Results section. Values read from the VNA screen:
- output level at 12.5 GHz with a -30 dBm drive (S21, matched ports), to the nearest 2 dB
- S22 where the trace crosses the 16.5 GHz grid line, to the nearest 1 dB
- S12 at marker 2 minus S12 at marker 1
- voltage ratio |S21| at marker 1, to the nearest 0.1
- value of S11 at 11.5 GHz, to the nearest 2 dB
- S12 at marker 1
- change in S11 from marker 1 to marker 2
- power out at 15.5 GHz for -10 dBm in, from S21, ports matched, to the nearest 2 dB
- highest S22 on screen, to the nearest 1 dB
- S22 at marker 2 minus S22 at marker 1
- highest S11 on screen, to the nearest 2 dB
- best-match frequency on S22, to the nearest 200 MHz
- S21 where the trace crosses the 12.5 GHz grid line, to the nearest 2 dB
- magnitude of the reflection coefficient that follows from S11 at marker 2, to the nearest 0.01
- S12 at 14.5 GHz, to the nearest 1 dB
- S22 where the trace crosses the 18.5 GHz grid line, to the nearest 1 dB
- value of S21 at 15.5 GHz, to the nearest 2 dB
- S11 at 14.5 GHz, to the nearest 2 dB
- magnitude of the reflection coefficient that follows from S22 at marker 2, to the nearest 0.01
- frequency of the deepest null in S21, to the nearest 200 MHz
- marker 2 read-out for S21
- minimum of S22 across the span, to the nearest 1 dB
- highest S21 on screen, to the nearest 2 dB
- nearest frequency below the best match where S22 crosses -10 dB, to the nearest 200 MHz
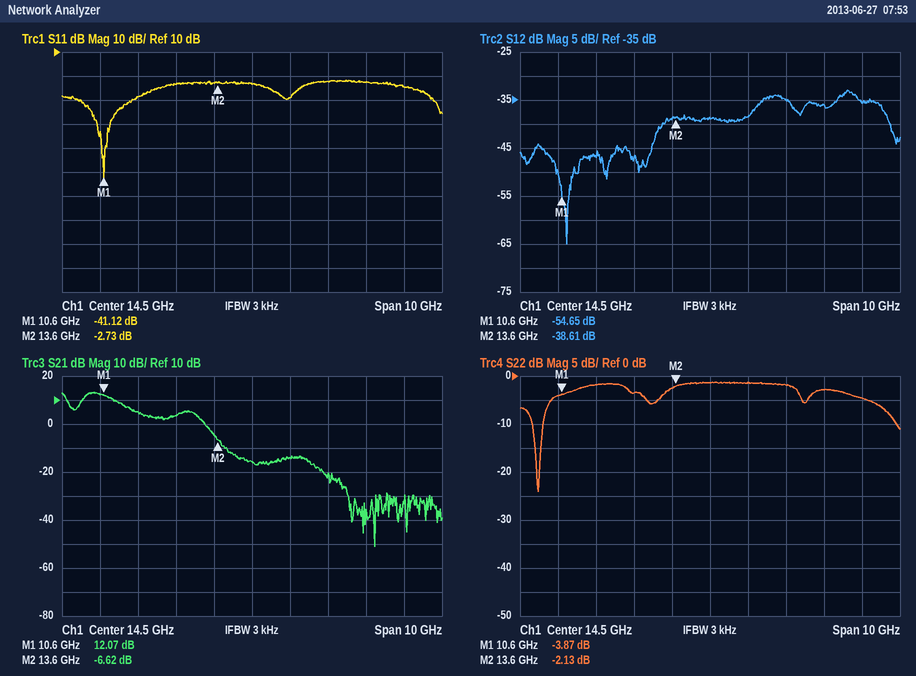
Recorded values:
-26 dBm
-2 dB
16.04 dB
4.0
-8 dB
-54.65 dB
38.39 dB
-24 dBm
-1 dB
1.74 dB
-2 dB
10.0 GHz
4 dB
0.73
-39 dB
-5 dB
-14 dB
-4 dB
0.78
17.8 GHz
-6.62 dB
-24 dB
14 dB
9.8 GHz
